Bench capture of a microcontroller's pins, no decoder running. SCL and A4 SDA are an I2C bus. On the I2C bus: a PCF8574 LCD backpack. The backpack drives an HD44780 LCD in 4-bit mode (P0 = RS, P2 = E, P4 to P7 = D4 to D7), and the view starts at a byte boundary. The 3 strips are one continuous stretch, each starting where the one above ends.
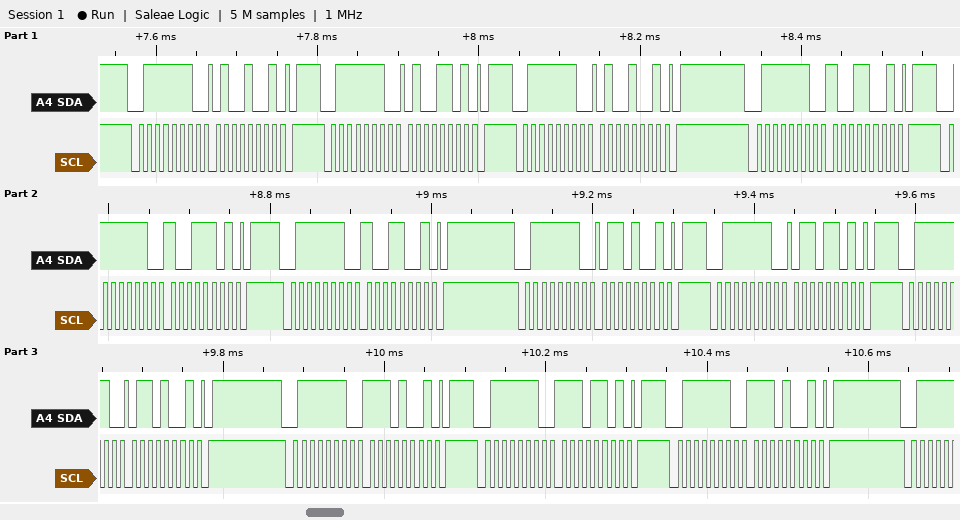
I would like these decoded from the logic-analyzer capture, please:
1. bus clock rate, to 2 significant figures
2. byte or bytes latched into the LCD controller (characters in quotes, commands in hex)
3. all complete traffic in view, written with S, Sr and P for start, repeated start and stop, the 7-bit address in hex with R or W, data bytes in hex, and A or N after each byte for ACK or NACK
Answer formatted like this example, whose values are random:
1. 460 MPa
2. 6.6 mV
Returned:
1. 100 kHz
2. 'I' 'n'
3. S 3FW A 49 A P S 3FW A 4D A P S 3FW A 49 A P S 3FW A 99 A P S 3FW A 9D A P S 3FW A 99 A P S 3FW A 69 A P S 3FW A 6D A P S 3FW A 69 A P S 3FW A E9 A P S 3FW A ED A P S 3FW A E9 A P
